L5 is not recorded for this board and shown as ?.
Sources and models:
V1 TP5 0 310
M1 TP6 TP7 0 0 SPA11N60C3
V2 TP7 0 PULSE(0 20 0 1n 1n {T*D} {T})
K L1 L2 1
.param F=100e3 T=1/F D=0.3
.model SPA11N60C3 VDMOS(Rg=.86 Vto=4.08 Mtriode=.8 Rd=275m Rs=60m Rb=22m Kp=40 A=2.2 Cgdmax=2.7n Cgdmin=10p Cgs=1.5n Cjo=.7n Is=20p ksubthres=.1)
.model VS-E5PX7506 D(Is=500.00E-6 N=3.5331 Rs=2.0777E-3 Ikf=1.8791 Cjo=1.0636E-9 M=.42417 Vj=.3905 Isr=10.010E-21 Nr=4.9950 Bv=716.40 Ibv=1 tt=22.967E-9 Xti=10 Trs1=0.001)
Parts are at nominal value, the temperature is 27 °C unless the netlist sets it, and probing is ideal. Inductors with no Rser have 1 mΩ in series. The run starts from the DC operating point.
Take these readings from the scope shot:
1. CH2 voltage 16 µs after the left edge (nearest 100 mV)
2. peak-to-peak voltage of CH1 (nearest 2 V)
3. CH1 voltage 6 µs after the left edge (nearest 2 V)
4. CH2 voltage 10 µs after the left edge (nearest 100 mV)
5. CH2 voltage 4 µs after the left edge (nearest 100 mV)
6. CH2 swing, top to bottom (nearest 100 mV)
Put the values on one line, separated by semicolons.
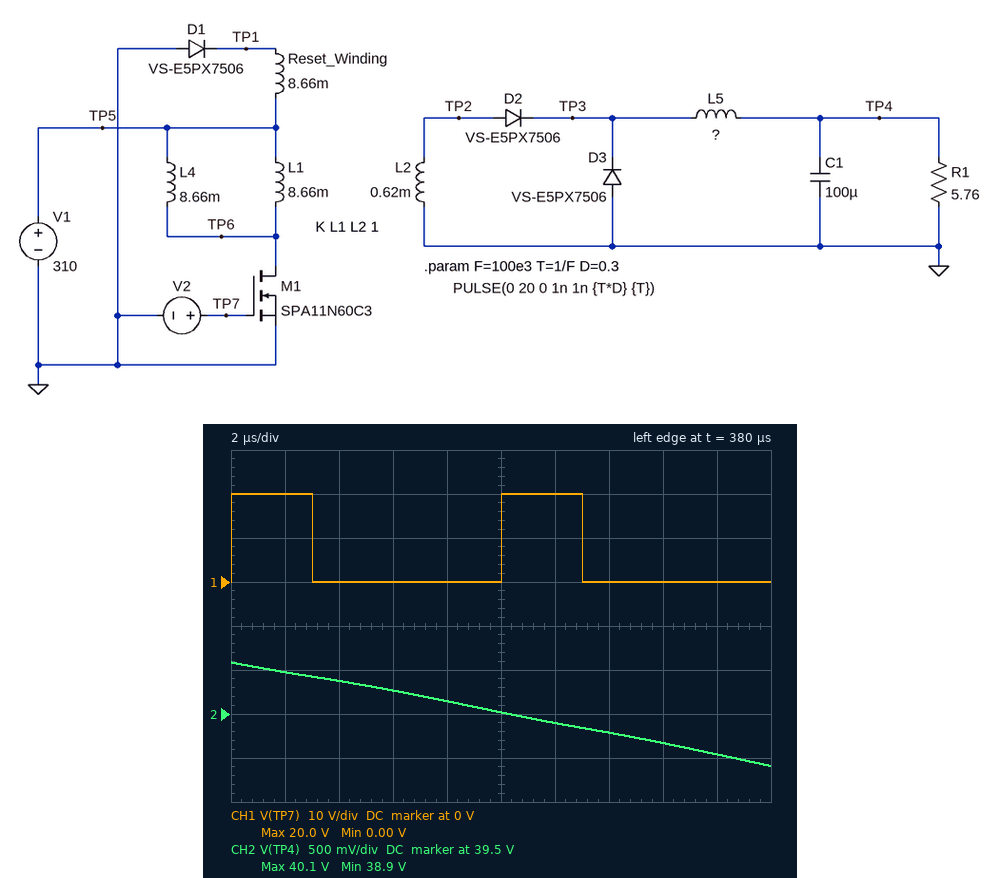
39.2 V; 20 V; 0 V; 39.5 V; 39.9 V; 1.2 V
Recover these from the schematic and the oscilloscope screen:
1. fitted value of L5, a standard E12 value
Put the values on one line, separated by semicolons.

120 µH
